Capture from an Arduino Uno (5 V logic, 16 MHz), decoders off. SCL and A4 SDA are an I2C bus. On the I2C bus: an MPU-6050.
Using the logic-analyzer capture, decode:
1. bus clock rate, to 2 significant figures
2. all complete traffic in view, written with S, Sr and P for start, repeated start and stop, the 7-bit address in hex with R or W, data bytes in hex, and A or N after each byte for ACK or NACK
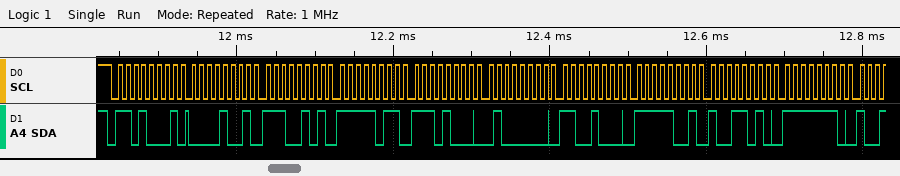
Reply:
100 kHz
S 68R A 09 A E5 A FB A E8 A 40 A C8 A F9 A 9A A FE A
